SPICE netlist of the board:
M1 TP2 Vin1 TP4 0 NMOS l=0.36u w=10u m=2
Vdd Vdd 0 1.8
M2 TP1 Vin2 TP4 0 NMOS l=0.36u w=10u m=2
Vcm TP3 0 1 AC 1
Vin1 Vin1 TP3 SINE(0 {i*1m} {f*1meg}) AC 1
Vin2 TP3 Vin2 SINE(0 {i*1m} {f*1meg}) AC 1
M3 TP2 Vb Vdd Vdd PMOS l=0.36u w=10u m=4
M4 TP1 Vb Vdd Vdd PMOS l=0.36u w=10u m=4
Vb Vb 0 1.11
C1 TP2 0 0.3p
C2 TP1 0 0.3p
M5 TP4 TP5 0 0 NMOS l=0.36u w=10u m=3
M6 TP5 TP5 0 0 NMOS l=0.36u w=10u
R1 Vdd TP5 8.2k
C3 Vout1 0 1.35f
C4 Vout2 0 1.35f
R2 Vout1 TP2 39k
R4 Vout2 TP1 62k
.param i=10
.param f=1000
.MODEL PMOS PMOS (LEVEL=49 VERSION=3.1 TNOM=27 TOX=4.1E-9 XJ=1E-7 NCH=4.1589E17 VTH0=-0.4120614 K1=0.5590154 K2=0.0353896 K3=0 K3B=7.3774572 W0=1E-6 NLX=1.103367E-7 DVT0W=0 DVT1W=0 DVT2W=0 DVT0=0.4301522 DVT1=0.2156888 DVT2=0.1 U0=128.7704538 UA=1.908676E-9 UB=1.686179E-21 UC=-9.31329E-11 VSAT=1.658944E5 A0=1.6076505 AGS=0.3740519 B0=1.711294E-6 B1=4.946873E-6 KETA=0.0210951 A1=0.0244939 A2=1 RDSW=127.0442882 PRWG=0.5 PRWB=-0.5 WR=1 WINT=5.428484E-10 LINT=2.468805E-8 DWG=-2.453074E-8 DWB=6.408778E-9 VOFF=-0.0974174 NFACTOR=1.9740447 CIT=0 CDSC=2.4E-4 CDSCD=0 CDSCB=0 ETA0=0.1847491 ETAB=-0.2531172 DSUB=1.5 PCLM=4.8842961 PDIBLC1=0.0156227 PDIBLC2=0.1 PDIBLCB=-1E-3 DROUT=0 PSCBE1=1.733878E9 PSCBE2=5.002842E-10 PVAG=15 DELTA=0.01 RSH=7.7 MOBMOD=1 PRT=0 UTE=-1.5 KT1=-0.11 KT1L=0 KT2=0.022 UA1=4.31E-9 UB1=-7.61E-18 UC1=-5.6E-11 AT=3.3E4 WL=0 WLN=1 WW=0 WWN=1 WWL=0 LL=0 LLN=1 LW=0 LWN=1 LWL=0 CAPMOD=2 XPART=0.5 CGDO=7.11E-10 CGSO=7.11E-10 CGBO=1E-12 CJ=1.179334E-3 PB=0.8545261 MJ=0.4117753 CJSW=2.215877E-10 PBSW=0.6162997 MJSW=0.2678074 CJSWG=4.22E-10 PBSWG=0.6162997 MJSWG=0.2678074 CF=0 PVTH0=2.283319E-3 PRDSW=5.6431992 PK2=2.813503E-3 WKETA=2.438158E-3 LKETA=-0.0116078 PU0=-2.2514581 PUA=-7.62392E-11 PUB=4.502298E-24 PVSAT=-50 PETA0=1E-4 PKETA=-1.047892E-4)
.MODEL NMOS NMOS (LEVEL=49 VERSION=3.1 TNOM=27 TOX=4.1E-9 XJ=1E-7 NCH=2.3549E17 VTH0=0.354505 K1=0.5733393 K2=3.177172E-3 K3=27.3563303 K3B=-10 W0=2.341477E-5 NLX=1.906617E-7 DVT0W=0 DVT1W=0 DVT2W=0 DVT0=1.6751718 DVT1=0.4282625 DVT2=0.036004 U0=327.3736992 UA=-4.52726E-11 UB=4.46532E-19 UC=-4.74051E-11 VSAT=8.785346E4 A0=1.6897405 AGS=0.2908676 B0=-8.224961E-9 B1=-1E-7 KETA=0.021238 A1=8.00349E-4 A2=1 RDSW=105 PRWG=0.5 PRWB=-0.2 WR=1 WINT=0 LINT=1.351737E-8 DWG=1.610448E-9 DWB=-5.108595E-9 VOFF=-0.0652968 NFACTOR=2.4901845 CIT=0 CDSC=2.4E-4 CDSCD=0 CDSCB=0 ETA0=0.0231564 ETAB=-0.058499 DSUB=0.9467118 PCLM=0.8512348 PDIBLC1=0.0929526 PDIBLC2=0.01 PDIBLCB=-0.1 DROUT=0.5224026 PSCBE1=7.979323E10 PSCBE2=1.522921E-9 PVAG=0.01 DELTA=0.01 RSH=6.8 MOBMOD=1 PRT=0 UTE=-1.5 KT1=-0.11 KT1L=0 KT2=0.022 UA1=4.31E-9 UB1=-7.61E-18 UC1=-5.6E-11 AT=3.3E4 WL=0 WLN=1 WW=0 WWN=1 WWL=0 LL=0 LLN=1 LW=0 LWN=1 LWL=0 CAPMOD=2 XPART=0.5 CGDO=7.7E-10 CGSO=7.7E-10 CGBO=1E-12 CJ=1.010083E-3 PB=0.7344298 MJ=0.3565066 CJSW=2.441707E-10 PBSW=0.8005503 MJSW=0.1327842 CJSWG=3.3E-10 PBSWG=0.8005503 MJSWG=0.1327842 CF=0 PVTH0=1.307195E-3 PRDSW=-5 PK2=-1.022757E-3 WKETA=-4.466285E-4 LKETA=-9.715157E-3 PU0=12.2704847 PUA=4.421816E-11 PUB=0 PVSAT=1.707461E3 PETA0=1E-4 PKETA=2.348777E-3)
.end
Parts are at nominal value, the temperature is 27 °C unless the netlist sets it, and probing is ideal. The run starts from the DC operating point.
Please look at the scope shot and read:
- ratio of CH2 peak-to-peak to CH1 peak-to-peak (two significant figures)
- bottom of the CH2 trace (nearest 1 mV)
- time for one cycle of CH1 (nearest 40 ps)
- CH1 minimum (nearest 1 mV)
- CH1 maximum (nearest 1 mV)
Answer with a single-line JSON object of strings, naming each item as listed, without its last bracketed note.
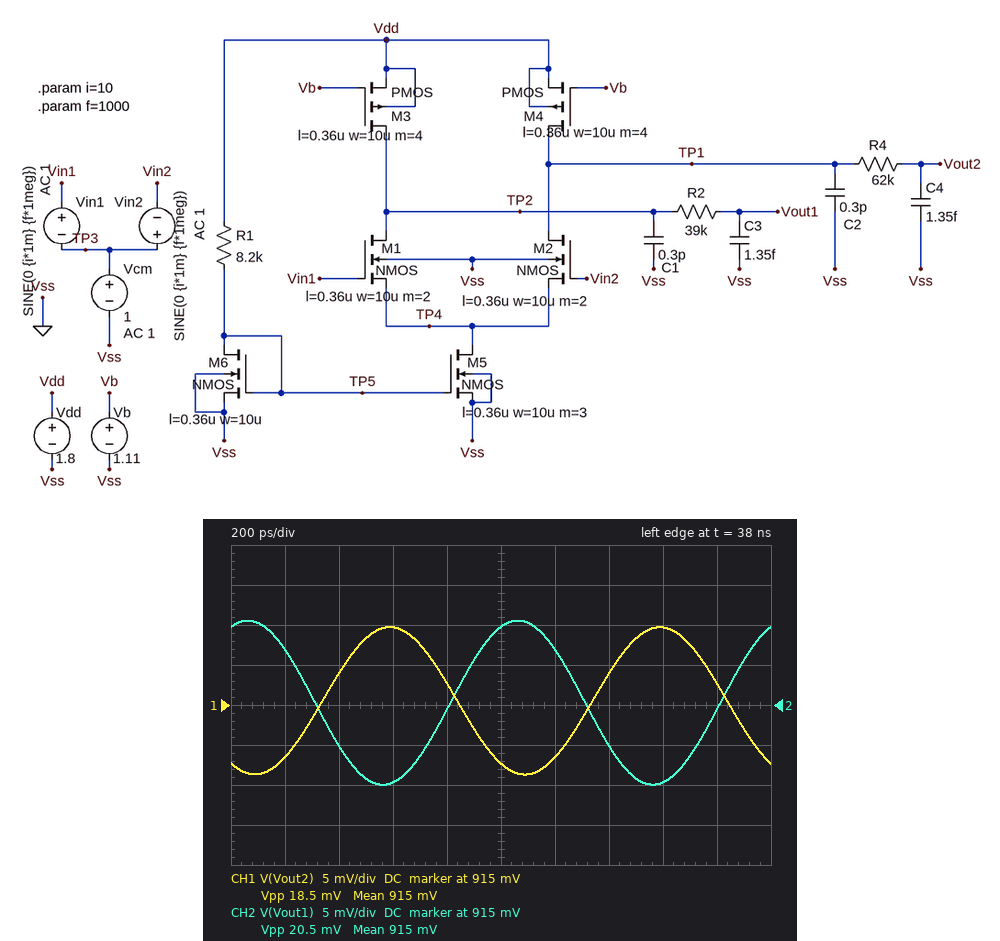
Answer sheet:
{"ratio of CH2 peak-to-peak to CH1 peak-to-peak": "1.1", "bottom of the CH2 trace": "905 mV", "time for one cycle of CH1": "1.00 ns", "CH1 minimum": "906 mV", "CH1 maximum": "925 mV"}
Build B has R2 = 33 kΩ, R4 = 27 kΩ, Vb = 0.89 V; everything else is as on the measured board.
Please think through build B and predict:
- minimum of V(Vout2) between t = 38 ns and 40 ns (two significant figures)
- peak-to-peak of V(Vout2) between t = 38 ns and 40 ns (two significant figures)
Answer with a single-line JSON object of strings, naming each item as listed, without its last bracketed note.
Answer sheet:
{"minimum of V(Vout2) between t = 38 ns and 40 ns": "1.7 V", "peak-to-peak of V(Vout2) between t = 38 ns and 40 ns": "12 mV"}
